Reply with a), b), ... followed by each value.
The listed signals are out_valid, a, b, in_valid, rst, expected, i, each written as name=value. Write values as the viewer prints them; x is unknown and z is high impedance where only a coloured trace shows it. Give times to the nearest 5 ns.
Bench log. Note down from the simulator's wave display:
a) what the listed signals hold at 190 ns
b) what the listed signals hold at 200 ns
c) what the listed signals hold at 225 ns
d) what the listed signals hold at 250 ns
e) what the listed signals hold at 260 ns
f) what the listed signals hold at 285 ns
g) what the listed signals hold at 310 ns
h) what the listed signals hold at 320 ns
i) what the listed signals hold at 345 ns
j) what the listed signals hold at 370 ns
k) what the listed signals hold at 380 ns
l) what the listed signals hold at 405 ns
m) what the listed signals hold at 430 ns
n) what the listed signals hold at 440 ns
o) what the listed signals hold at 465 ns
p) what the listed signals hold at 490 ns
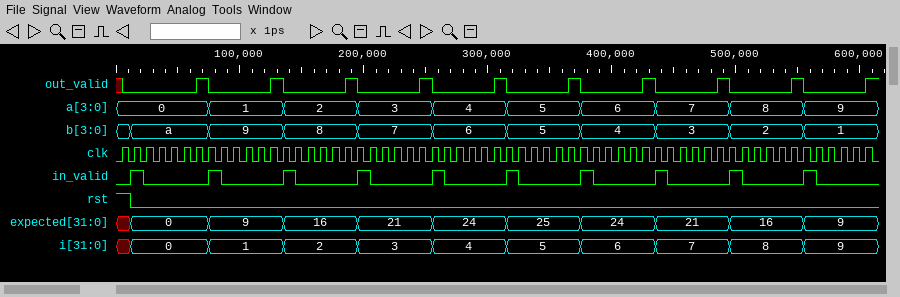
a) out_valid=1, a=2, b=8, in_valid=0, rst=0, expected=16, i=2
b) out_valid=0, a=3, b=7, in_valid=1, rst=0, expected=21, i=3
c) out_valid=0, a=3, b=7, in_valid=0, rst=0, expected=21, i=3
d) out_valid=1, a=3, b=7, in_valid=0, rst=0, expected=21, i=3
e) out_valid=0, a=4, b=6, in_valid=1, rst=0, expected=24, i=4
f) out_valid=0, a=4, b=6, in_valid=0, rst=0, expected=24, i=4
g) out_valid=1, a=4, b=6, in_valid=0, rst=0, expected=24, i=4
h) out_valid=0, a=5, b=5, in_valid=1, rst=0, expected=25, i=5
i) out_valid=0, a=5, b=5, in_valid=0, rst=0, expected=25, i=5
j) out_valid=1, a=5, b=5, in_valid=0, rst=0, expected=25, i=5
k) out_valid=0, a=6, b=4, in_valid=1, rst=0, expected=24, i=6
l) out_valid=0, a=6, b=4, in_valid=0, rst=0, expected=24, i=6
m) out_valid=1, a=6, b=4, in_valid=0, rst=0, expected=24, i=6
n) out_valid=0, a=7, b=3, in_valid=1, rst=0, expected=21, i=7
o) out_valid=0, a=7, b=3, in_valid=0, rst=0, expected=21, i=7
p) out_valid=1, a=7, b=3, in_valid=0, rst=0, expected=21, i=7
